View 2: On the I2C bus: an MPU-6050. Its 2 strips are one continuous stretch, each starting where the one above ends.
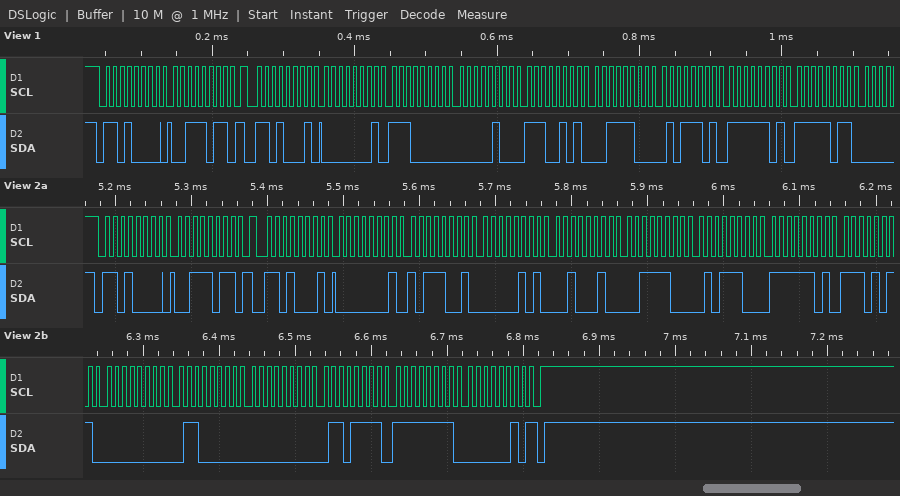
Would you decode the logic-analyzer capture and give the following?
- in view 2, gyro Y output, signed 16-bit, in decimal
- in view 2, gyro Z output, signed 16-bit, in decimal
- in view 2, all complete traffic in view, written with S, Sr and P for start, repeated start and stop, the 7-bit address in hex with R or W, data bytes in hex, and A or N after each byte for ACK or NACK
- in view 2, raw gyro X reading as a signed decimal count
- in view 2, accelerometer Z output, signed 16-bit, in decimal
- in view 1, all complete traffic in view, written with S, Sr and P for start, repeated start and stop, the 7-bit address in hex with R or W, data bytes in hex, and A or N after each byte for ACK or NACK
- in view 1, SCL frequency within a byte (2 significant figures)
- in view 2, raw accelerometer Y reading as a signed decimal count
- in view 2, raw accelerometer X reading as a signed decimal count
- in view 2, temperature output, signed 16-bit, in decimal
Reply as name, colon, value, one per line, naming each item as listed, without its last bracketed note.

in view 2, gyro Y output, signed 16-bit, in decimal: 111
in view 2, gyro Z output, signed 16-bit, in decimal: -254
in view 2, all complete traffic in view, written with S, Sr and P for start, repeated start and stop, the 7-bit address in hex with R or W, data bytes in hex, and A or N after each byte for ACK or NACK: S 68W A 3B A Sr 68R A 01 A B9 A 05 A 22 A 3C A 5C A FD A EB A 00 A 60 A 00 A 6F A FF A 02 N P
in view 2, raw gyro X reading as a signed decimal count: 96
in view 2, accelerometer Z output, signed 16-bit, in decimal: 15452
in view 1, all complete traffic in view, written with S, Sr and P for start, repeated start and stop, the 7-bit address in hex with R or W, data bytes in hex, and A or N after each byte for ACK or NACK: S 68W A 3B A Sr 68R A 01 A E0 A 04 A E5 A 3C A 5D A FD A FB A
in view 1, SCL frequency within a byte: 100 kHz
in view 2, raw accelerometer Y reading as a signed decimal count: 1314
in view 2, raw accelerometer X reading as a signed decimal count: 441
in view 2, temperature output, signed 16-bit, in decimal: -533
